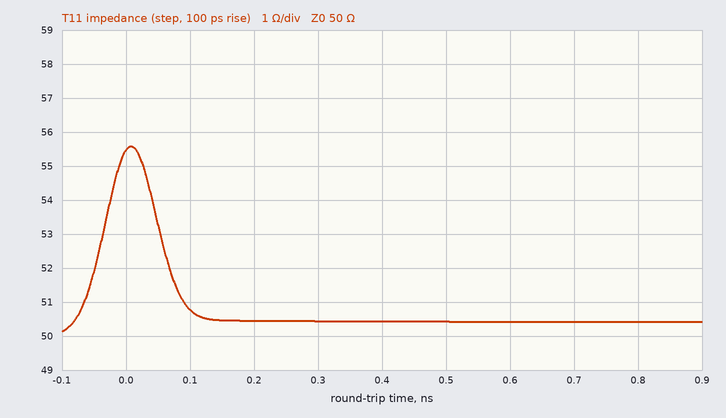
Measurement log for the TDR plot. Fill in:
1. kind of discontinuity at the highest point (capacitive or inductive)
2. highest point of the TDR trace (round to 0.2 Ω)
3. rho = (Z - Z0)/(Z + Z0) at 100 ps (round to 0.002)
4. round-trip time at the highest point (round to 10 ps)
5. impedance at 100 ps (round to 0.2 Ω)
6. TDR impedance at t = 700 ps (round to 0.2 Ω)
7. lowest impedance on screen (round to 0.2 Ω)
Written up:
inductive
55.6 Ω
+0.008
10 ps
50.8 Ω
50.4 Ω
50.2 Ω
